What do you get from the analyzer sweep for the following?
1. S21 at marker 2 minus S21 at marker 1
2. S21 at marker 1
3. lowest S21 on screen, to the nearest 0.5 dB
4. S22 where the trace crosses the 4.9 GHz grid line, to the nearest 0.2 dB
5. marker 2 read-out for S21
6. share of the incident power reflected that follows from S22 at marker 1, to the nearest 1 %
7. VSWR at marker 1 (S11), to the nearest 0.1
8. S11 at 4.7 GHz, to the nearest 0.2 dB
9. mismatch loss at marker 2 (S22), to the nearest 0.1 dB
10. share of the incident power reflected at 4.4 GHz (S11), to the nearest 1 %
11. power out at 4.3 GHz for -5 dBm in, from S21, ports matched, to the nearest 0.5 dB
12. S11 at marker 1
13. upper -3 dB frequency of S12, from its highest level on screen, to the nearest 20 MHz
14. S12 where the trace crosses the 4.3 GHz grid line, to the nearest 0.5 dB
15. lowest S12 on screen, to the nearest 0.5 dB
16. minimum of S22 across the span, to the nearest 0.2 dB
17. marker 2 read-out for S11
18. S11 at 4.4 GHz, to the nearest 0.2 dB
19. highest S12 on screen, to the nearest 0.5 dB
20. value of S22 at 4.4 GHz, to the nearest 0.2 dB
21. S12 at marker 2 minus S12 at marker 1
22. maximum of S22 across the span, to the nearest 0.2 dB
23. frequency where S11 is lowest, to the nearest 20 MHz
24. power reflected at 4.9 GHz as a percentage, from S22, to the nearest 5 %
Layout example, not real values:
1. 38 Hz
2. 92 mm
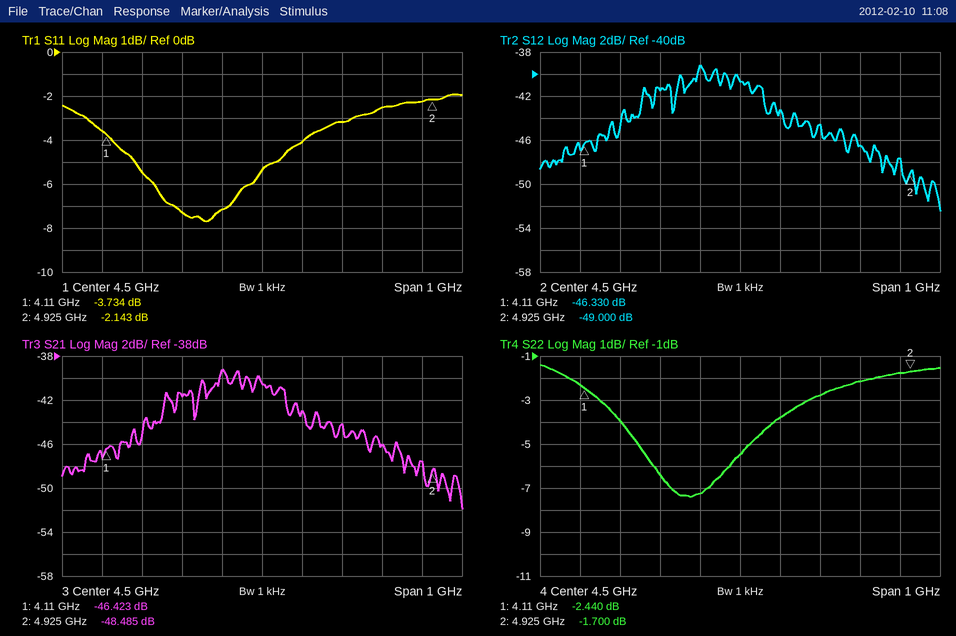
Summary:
1. -2.062 dB
2. -46.423 dB
3. -52.0 dB
4. -1.8 dB
5. -48.485 dB
6. 57 %
7. 4.7
8. -3.2 dB
9. 4.9 dB
10. 19 %
11. -46.5 dBm
12. -3.734 dB
13. 4.56 GHz
14. -41.5 dB
15. -52.5 dB
16. -7.4 dB
17. -2.143 dB
18. -7.2 dB
19. -39.0 dB
20. -7.2 dB
21. -2.670 dB
22. -1.4 dB
23. 4.36 GHz
24. 65 %
